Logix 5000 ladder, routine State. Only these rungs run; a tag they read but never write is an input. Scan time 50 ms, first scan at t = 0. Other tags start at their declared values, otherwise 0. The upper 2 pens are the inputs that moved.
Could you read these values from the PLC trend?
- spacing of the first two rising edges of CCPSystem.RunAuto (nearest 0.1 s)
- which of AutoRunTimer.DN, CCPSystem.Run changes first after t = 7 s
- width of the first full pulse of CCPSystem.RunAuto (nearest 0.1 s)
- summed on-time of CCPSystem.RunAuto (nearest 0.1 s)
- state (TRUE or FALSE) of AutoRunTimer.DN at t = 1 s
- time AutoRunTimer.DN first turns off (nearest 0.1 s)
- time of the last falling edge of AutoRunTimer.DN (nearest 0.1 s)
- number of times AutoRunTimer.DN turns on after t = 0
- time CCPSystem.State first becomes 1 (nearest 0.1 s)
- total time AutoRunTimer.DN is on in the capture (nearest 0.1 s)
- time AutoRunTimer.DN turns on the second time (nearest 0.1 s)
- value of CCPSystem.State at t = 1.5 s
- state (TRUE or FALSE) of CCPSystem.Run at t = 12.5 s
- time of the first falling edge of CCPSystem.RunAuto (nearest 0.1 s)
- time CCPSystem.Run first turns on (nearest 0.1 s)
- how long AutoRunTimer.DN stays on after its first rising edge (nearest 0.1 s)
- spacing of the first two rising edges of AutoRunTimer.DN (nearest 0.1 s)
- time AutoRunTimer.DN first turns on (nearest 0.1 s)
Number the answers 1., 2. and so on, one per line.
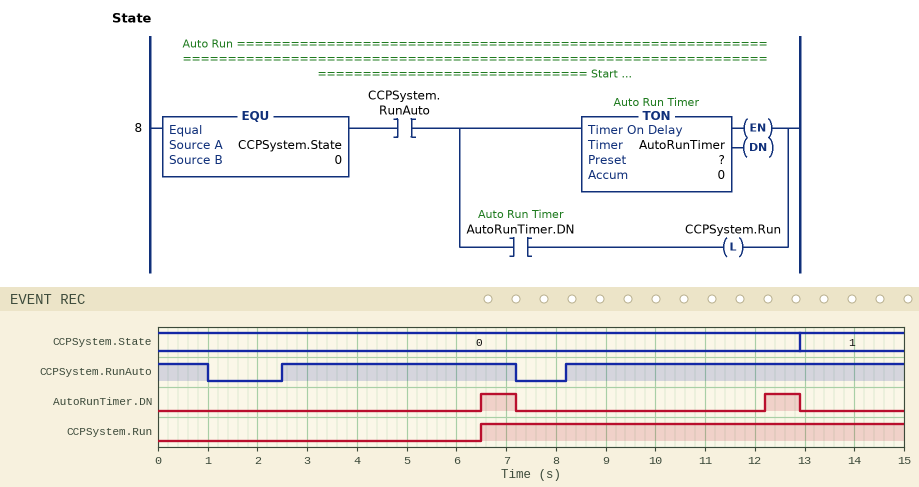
1. 5.7 s
2. AutoRunTimer.DN
3. 4.7 s
4. 12.5 s
5. FALSE
6. 7.2 s
7. 12.9 s
8. 2
9. 12.9 s
10. 1.4 s
11. 12.2 s
12. 0
13. TRUE
14. 1.0 s
15. 6.5 s
16. 0.7 s
17. 5.7 s
18. 6.5 s
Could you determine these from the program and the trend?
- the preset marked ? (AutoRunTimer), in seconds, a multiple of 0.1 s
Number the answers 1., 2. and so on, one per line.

1. 4.0 s
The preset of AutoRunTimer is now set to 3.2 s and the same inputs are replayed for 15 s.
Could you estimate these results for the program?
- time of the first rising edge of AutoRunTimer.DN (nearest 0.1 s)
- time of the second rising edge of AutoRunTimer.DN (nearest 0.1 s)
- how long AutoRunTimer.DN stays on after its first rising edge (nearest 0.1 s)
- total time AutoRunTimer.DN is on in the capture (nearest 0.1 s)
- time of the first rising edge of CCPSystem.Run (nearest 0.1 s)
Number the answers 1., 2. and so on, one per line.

1. 5.7 s
2. 11.4 s
3. 1.5 s
4. 3.0 s
5. 5.7 s
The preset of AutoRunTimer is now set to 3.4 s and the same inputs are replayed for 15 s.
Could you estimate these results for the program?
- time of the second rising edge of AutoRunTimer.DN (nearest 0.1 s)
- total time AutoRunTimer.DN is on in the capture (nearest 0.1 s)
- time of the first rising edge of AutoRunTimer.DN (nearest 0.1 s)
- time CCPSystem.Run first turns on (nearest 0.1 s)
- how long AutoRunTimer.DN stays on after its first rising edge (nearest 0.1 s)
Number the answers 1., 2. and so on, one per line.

1. 11.6 s
2. 2.6 s
3. 5.9 s
4. 5.9 s
5. 1.3 s
